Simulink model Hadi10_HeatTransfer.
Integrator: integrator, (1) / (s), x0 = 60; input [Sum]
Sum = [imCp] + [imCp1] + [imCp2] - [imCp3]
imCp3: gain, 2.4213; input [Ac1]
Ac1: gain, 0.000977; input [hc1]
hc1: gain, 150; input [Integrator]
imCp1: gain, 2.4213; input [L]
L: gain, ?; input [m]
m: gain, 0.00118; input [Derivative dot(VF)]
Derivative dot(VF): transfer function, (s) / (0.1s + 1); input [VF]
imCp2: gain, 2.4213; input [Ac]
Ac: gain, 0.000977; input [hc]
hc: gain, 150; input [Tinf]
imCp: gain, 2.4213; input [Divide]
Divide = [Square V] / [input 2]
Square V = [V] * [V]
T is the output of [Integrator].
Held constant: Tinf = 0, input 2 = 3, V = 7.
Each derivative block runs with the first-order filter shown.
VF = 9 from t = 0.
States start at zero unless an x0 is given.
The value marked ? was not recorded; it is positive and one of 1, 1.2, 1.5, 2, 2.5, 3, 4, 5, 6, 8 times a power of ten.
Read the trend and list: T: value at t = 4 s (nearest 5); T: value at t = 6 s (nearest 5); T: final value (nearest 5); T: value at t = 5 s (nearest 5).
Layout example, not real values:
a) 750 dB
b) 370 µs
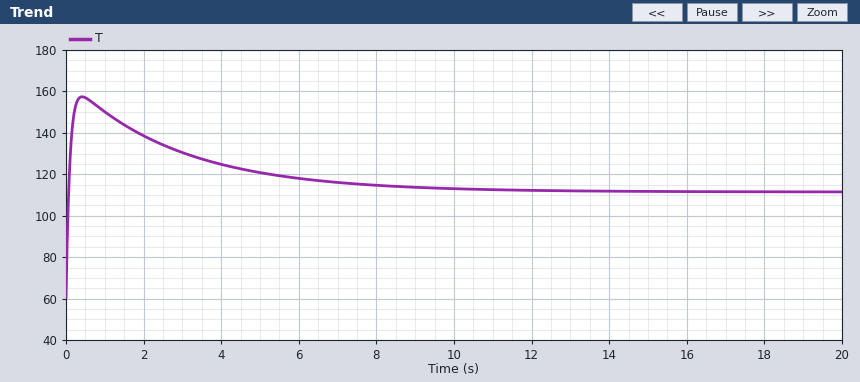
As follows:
a) 125
b) 120
c) 110
d) 120
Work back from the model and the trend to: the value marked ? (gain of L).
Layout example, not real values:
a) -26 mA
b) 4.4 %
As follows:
a) 4000
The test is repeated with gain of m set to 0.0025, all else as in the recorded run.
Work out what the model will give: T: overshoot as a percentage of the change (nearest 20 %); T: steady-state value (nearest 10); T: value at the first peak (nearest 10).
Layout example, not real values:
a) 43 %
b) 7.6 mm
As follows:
a) 280 %
b) 110
c) 260
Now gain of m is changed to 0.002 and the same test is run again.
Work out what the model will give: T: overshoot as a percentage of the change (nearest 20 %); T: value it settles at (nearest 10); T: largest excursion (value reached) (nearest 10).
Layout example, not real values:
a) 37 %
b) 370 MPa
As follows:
a) 220 %
b) 110
c) 220
